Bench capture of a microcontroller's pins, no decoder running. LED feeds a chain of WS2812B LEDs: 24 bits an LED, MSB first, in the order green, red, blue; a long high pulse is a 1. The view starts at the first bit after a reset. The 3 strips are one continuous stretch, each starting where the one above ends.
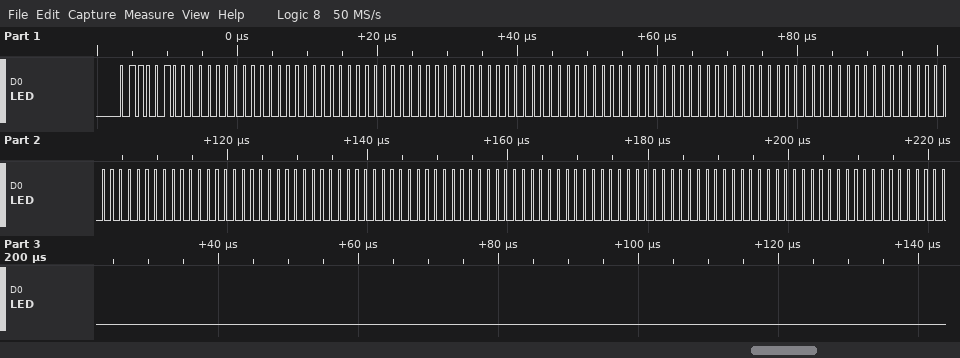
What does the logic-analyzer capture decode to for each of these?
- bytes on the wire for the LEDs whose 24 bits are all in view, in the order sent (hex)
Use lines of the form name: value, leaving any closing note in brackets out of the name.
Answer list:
bytes on the wire for the LEDs whose 24 bits are all in view, in the order sent: 64 00 00 00 00 00 00 00 00 00 00 00 00 00 00 00 00 00 00 00 00 00 00 00
